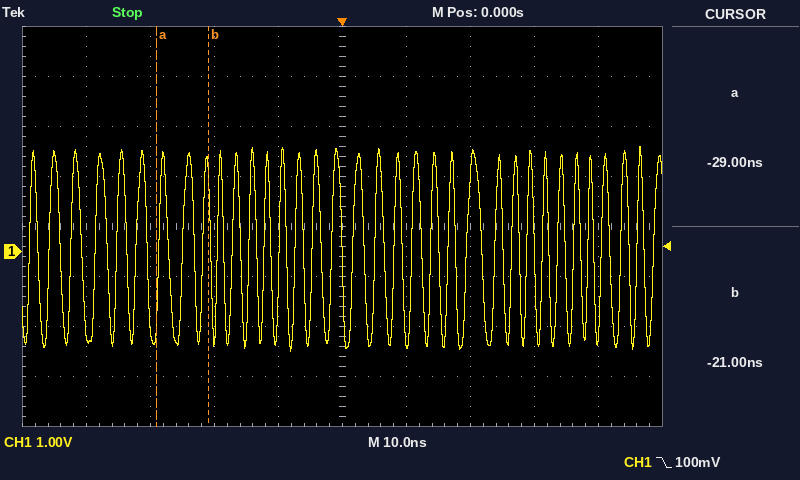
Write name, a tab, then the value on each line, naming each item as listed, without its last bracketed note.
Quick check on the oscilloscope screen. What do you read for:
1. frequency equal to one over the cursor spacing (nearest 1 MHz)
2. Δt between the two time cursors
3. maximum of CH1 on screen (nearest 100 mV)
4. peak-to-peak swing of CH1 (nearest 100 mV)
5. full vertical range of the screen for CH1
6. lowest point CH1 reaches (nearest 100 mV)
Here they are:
frequency equal to one over the cursor spacing	125 MHz
Δt between the two time cursors	8 ns
maximum of CH1 on screen	2.1 V
peak-to-peak swing of CH1	4.1 V
full vertical range of the screen for CH1	8 V
lowest point CH1 reaches	-2.0 V
